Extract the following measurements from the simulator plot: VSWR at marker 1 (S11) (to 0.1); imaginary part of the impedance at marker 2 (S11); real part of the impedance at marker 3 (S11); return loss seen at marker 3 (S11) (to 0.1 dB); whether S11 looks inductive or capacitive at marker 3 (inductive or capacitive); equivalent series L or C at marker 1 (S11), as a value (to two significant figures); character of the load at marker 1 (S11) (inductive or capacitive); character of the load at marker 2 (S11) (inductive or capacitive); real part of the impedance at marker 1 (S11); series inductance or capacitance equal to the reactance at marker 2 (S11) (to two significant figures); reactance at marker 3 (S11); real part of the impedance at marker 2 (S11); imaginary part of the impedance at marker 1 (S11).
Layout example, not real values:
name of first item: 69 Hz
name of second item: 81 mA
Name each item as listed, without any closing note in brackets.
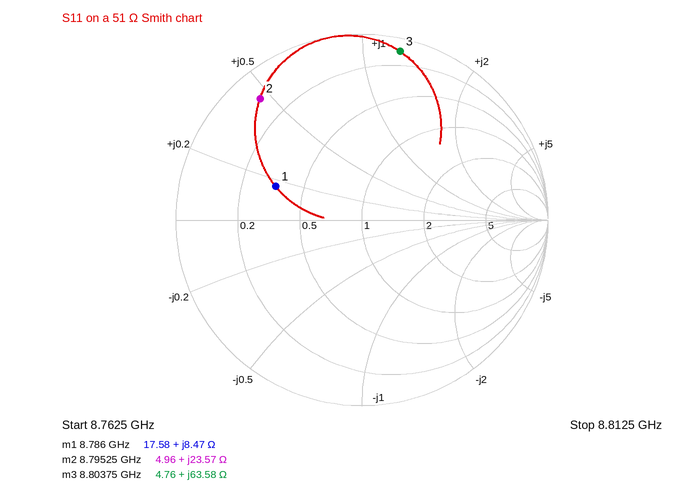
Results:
VSWR at marker 1 (S11): 3.0
imaginary part of the impedance at marker 2: +23.57 Ω
real part of the impedance at marker 3: 4.76 Ω
return loss seen at marker 3 (S11): 0.6 dB
whether S11 looks inductive or capacitive at marker 3: inductive
equivalent series L or C at marker 1 (S11), as a value: 150 pH
character of the load at marker 1 (S11): inductive
character of the load at marker 2 (S11): inductive
real part of the impedance at marker 1: 17.58 Ω
series inductance or capacitance equal to the reactance at marker 2 (S11): 430 pH
reactance at marker 3: +63.58 Ω
real part of the impedance at marker 2: 4.96 Ω
imaginary part of the impedance at marker 1: +8.47 Ω
